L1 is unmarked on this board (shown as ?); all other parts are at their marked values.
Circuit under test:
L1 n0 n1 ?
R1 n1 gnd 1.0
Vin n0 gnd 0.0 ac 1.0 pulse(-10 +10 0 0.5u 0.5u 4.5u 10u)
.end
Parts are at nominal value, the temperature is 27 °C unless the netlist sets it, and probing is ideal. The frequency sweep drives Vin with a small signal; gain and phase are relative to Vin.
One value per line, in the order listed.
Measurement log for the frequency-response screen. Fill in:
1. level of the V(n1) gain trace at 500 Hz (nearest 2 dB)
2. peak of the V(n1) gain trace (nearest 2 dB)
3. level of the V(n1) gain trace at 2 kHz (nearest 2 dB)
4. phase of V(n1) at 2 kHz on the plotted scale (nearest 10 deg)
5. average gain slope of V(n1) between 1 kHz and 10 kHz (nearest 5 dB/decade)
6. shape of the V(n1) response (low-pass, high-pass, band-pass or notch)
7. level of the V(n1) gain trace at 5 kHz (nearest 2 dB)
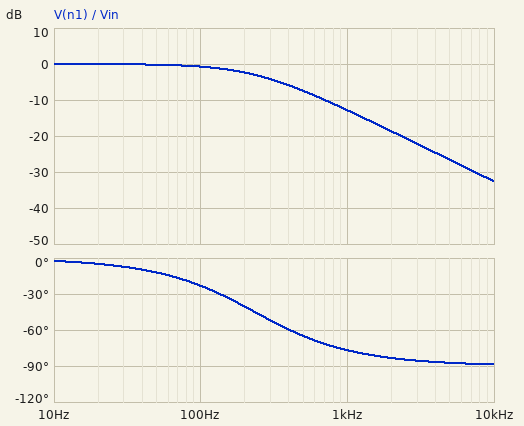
-8 dB
0 dB
-18 dB
-80 deg
-20 dB/decade
low-pass
-26 dB
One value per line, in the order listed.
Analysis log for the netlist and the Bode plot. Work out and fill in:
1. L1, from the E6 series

680 µH
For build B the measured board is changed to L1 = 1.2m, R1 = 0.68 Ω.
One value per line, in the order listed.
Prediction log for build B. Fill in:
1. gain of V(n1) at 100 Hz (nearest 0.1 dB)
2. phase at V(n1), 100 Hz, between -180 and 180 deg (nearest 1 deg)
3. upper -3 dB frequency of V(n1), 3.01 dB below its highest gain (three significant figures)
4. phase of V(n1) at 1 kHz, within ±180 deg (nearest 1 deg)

-3.5 dB
-48 deg
90.2 Hz
-85 deg
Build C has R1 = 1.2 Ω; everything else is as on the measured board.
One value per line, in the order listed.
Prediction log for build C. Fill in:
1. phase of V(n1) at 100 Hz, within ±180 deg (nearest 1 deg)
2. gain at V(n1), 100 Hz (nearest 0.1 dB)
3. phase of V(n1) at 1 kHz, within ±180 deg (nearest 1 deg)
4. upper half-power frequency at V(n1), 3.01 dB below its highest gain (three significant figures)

-20 deg
-0.5 dB
-74 deg
281 Hz
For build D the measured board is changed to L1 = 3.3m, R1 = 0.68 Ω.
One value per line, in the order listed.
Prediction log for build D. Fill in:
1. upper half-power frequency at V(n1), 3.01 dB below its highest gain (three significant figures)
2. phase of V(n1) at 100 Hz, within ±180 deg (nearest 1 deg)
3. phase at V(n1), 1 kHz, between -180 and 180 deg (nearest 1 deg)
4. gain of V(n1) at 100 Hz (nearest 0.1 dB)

32.8 Hz
-72 deg
-88 deg
-10.1 dB
